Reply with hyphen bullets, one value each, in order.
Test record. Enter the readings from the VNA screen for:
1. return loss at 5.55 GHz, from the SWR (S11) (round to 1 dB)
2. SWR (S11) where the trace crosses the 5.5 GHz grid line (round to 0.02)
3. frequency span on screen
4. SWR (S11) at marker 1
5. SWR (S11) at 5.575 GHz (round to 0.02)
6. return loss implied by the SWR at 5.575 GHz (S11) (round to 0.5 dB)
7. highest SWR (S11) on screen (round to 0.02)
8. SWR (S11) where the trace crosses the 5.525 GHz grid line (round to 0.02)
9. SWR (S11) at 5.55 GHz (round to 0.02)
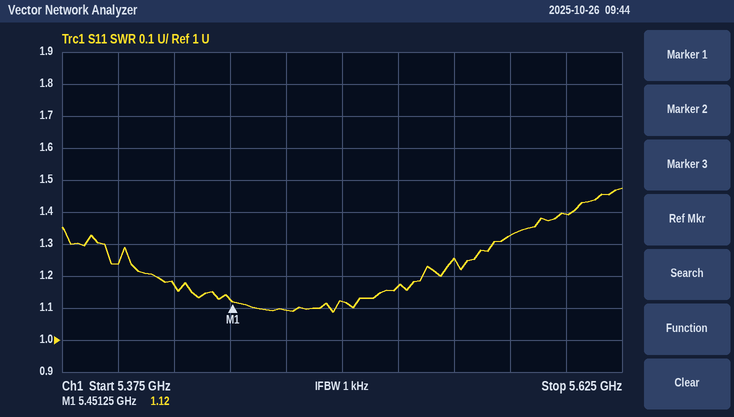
- 19 dB
- 1.12
- 250 MHz
- 1.12
- 1.32
- 17.0 dB
- 1.48
- 1.16
- 1.26
